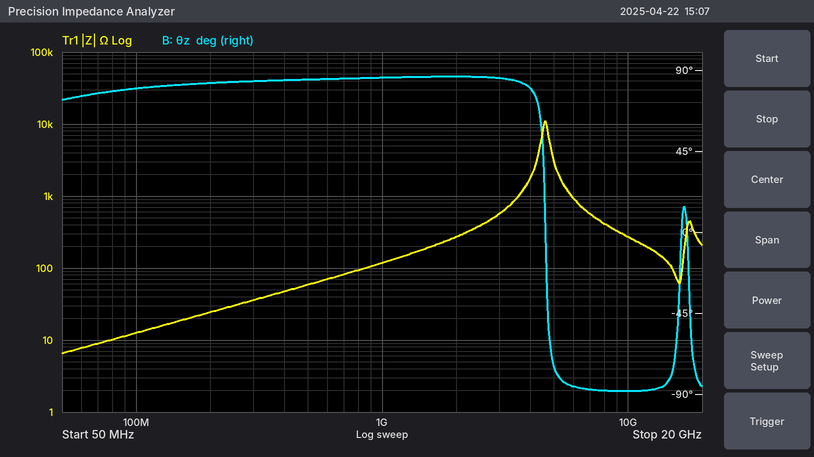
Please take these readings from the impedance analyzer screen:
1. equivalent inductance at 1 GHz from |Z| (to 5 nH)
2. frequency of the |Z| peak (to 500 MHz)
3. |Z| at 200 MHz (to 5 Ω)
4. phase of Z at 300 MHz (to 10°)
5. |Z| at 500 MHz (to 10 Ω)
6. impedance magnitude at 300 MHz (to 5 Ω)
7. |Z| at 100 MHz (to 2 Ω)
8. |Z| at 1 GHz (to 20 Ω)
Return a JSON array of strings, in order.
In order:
["20 nH", "4.5 GHz", "25 Ω", "80°", "60 Ω", "35 Ω", "12 Ω", "120 Ω"]
